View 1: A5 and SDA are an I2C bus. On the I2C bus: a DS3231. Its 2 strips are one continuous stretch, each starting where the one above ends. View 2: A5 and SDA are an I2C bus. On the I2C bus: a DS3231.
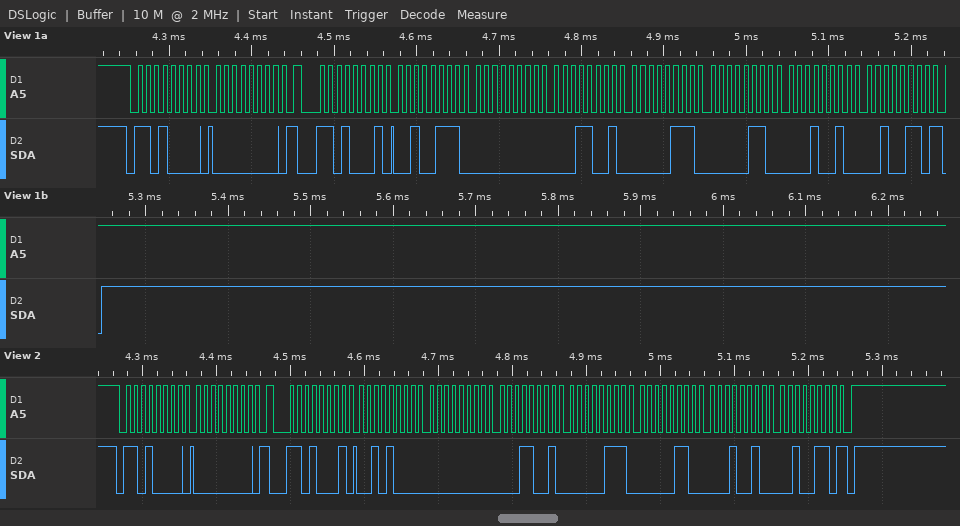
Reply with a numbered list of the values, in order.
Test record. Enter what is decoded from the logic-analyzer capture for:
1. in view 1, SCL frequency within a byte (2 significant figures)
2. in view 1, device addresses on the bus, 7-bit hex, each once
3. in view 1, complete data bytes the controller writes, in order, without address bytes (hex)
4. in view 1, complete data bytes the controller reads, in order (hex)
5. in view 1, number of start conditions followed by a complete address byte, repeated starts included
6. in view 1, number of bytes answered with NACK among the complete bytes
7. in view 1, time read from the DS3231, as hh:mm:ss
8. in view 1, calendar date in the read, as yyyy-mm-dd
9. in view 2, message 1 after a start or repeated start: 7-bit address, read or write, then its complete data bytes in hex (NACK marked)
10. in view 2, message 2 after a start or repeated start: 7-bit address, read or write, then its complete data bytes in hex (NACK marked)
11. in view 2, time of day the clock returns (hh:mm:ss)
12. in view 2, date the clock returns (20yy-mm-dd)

1. 100 kHz
2. 0x68
3. 00
4. 27 00 19 07 06 12 26
5. 2
6. 1
7. 19:00:27
8. 2026-12-06
9. 0x68 write: 00
10. 0x68 read: 28 00 19 07 06 12 26 NACK
11. 19:00:28
12. 2026-12-06
